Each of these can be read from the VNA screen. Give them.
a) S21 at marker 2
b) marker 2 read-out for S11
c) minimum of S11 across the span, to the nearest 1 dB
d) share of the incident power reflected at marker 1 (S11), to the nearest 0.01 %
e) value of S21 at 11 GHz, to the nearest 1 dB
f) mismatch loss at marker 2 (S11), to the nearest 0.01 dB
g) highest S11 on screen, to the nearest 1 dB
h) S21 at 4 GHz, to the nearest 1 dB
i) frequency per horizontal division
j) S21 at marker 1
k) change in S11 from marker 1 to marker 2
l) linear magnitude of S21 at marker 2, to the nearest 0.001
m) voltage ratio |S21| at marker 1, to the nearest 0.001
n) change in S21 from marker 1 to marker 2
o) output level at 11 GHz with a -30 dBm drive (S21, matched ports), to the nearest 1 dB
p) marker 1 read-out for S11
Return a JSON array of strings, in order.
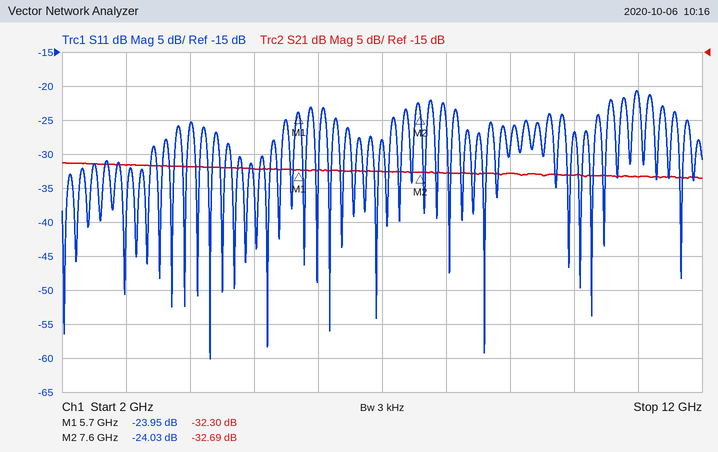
["-32.69 dB", "-24.03 dB", "-60 dB", "0.40 %", "-33 dB", "0.02 dB", "-21 dB", "-32 dB", "1 GHz", "-32.30 dB", "-0.08 dB", "0.023", "0.024", "-0.39 dB", "-63 dBm", "-23.95 dB"]
